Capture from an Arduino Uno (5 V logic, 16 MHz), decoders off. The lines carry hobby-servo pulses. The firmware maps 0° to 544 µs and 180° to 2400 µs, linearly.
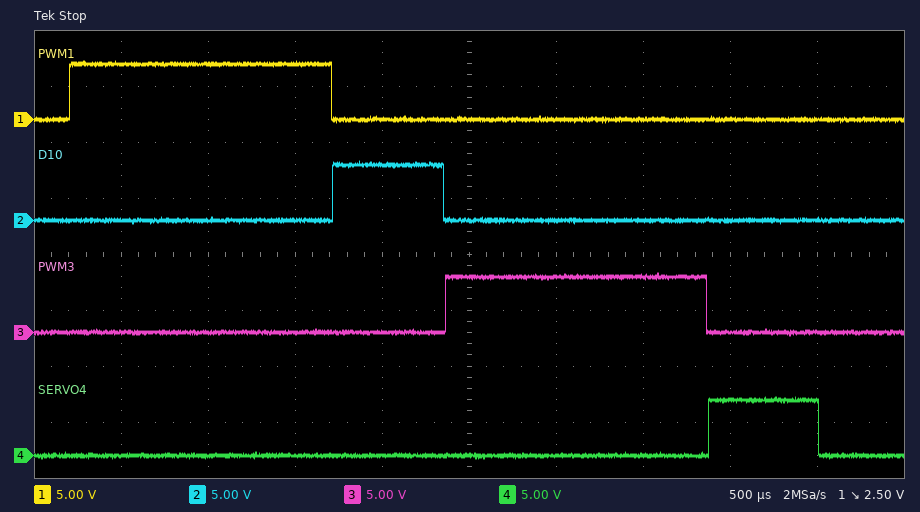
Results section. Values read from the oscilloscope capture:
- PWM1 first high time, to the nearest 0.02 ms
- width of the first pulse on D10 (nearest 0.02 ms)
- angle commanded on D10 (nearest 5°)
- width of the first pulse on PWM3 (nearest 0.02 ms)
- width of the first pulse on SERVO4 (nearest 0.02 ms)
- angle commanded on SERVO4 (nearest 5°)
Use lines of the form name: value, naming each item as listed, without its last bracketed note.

PWM1 first high time, to the nearest 0.02 ms: 1.50 ms
width of the first pulse on D10: 0.64 ms
angle commanded on D10: 10°
width of the first pulse on PWM3: 1.50 ms
width of the first pulse on SERVO4: 0.64 ms
angle commanded on SERVO4: 10°
